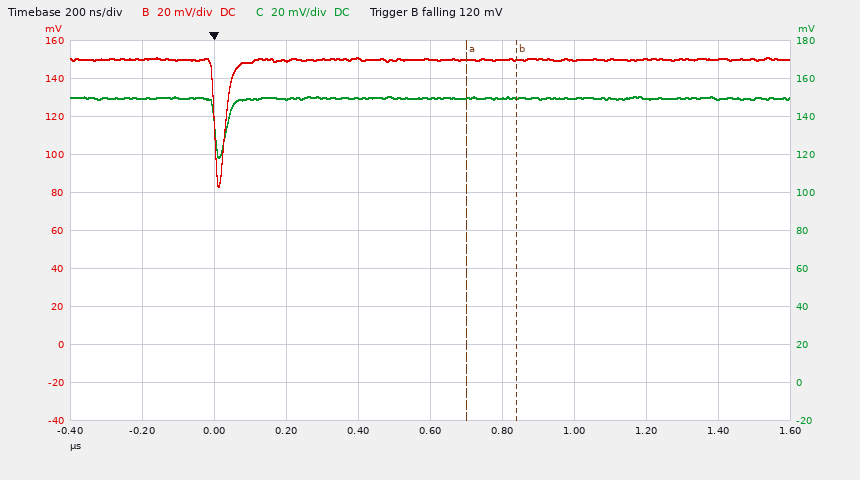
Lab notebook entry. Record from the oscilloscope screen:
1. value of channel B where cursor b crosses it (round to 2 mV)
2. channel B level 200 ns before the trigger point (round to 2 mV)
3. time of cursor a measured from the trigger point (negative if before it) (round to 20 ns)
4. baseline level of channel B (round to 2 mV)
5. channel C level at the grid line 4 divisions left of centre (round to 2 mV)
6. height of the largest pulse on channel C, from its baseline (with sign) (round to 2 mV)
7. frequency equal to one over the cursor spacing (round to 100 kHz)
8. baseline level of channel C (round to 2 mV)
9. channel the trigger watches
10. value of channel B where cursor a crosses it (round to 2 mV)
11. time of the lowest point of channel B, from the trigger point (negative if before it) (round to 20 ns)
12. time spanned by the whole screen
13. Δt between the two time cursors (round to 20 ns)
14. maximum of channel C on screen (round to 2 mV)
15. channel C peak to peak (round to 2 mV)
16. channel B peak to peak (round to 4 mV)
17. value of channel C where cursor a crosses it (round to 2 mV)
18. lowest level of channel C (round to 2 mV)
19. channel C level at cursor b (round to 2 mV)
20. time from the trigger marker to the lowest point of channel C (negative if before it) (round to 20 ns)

150 mV
150 mV
+700 ns
150 mV
150 mV
-32 mV
7.1 MHz
150 mV
channel B
150 mV
+20 ns
2 µs
140 ns
150 mV
32 mV
68 mV
150 mV
118 mV
150 mV
+20 ns
